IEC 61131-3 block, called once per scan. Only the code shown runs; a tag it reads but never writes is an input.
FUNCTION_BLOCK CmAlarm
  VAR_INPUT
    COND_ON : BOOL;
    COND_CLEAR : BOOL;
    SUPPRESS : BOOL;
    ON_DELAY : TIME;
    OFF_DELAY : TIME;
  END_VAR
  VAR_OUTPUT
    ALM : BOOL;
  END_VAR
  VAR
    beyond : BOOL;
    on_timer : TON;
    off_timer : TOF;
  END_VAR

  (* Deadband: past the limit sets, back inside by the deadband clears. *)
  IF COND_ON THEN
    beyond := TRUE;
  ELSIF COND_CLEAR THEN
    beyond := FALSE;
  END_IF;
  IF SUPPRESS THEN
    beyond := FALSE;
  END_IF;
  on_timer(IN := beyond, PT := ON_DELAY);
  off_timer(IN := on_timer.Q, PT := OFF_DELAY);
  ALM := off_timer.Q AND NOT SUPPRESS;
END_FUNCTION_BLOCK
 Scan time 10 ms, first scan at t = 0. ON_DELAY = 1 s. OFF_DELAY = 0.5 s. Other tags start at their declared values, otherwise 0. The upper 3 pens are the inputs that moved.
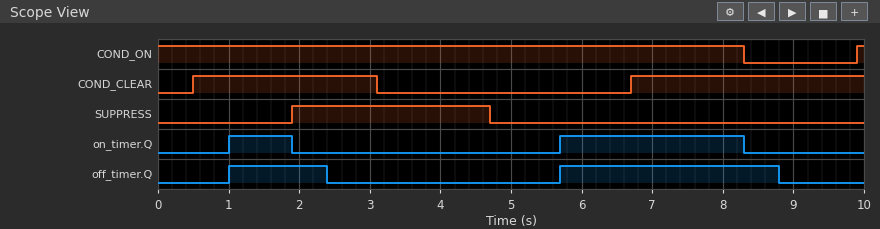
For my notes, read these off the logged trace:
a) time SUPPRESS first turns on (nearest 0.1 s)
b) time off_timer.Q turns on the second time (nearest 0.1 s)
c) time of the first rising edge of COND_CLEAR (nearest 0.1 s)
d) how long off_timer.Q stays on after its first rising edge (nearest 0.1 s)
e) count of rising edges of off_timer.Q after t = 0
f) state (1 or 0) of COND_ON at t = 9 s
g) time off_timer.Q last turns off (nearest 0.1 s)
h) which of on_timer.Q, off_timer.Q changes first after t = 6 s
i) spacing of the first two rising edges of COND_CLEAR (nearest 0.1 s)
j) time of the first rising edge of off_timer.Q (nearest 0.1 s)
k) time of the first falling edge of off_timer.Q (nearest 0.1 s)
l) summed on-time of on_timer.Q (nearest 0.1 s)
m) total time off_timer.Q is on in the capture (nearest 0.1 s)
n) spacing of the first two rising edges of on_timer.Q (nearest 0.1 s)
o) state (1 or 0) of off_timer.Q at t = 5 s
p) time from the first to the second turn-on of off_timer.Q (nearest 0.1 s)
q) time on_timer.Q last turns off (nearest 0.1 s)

1.9 s
5.7 s
0.5 s
1.4 s
2
0
8.8 s
on_timer.Q
6.2 s
1.0 s
2.4 s
3.5 s
4.5 s
4.7 s
0
4.7 s
8.3 s
